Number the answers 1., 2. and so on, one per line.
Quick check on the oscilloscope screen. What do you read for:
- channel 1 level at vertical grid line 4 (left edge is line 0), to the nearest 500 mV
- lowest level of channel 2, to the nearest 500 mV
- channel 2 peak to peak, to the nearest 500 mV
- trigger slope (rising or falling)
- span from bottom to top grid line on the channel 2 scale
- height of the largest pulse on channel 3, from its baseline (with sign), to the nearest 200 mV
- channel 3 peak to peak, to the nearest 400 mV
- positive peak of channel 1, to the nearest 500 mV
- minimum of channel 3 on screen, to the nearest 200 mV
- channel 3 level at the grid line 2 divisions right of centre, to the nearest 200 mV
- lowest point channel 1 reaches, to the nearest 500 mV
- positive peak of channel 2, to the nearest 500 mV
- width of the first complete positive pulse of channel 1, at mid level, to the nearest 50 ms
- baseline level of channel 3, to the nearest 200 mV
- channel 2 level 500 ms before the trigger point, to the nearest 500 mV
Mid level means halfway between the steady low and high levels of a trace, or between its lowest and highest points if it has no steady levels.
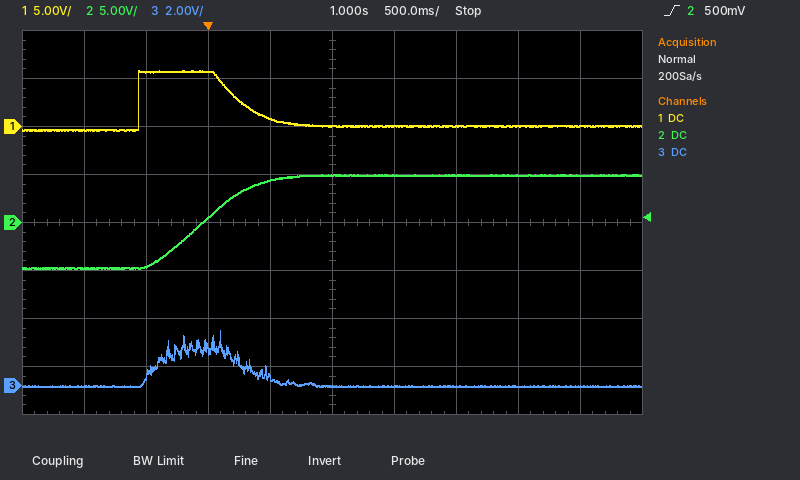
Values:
1. 1.0 V
2. -5.0 V
3. 10.0 V
4. rising
5. 40 V
6. +2.4 V
7. 2.4 V
8. 6.0 V
9. 0.0 V
10. 0.0 V
11. -500 mV
12. 5.0 V
13. 800 ms
14. 0.0 V
15. -4.5 V
